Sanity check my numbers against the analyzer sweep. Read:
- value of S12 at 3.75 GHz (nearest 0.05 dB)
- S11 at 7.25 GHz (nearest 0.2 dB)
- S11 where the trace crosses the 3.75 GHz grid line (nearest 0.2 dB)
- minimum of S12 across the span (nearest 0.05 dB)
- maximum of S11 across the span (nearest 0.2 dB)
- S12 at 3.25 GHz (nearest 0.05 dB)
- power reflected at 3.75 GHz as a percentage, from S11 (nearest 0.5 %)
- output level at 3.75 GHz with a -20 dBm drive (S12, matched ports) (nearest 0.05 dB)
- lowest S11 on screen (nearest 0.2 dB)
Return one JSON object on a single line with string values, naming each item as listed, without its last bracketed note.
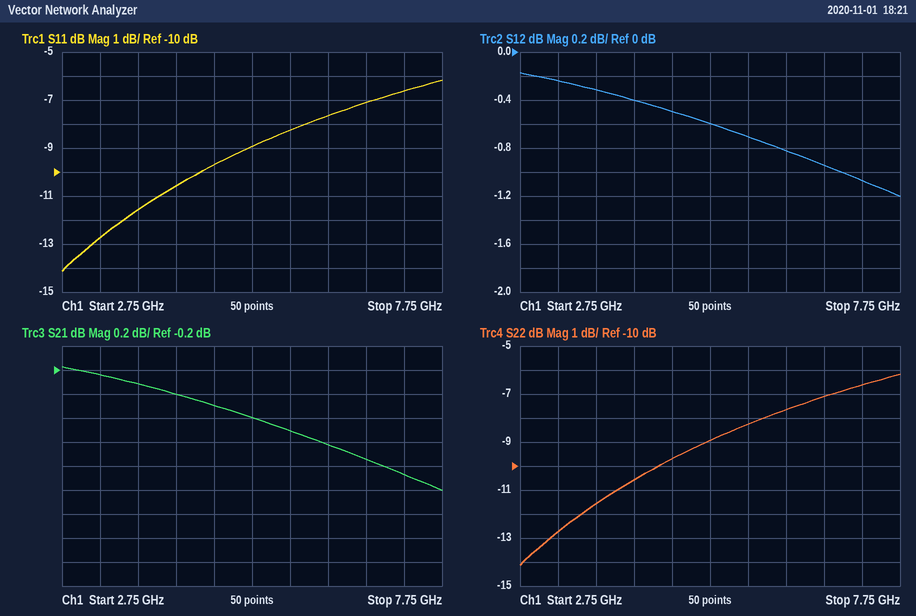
{"value of S12 at 3.75 GHz": "-0.30 dB", "S11 at 7.25 GHz": "-6.6 dB", "S11 where the trace crosses the 3.75 GHz grid line": "-11.6 dB", "minimum of S12 across the span": "-1.20 dB", "maximum of S11 across the span": "-6.2 dB", "S12 at 3.25 GHz": "-0.25 dB", "power reflected at 3.75 GHz as a percentage, from S11": "7.0 %", "output level at 3.75 GHz with a -20 dBm drive (S12, matched ports)": "-20.30 dBm", "lowest S11 on screen": "-14.2 dB"}
